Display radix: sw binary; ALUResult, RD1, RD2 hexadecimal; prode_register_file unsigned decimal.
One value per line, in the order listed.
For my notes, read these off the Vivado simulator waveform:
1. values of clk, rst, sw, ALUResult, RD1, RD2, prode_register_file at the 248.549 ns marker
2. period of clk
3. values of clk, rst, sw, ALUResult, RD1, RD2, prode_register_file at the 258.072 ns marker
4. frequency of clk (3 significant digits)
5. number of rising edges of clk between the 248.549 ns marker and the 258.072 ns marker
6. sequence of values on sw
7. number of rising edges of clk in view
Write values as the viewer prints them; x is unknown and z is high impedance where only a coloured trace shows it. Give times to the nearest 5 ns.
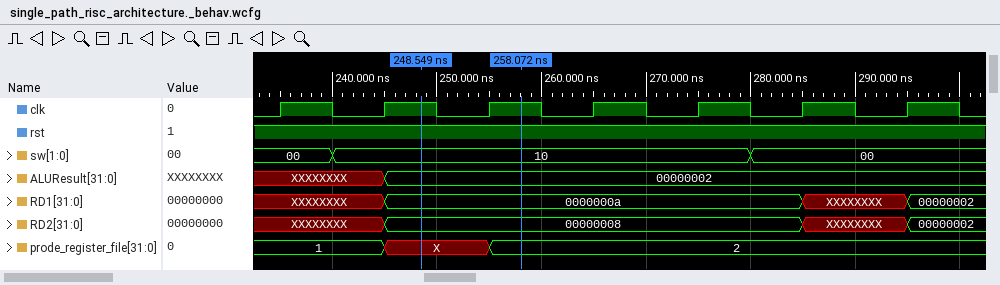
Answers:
clk=1, rst=1, sw=10, ALUResult=00000002, RD1=0000000a, RD2=00000008, prode_register_file=X
10 ns
clk=1, rst=1, sw=10, ALUResult=00000002, RD1=0000000a, RD2=00000008, prode_register_file=2
100 MHz
1
00, 10, 00
7
